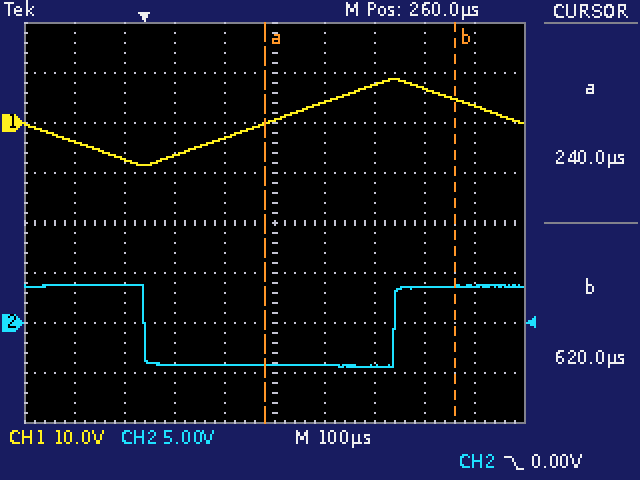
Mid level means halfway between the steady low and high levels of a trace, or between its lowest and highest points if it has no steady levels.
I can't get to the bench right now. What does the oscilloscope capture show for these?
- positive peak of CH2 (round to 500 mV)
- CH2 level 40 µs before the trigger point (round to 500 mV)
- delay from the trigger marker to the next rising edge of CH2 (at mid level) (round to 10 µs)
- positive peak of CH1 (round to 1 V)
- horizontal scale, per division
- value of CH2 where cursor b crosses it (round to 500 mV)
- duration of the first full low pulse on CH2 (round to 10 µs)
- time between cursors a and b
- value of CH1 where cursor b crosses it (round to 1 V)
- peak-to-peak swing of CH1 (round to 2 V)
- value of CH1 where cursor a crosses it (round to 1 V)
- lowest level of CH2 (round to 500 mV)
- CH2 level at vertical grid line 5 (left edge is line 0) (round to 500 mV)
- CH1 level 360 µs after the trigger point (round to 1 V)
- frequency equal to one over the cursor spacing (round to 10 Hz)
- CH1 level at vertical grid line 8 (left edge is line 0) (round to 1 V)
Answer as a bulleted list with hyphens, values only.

- 4.0 V
- 4.0 V
- 500 µs
- 9 V
- 100 µs
- 3.5 V
- 500 µs
- 380 µs
- 5 V
- 18 V
- 0 V
- -4.5 V
- -4.0 V
- 4 V
- 2.63 kHz
- 7 V
